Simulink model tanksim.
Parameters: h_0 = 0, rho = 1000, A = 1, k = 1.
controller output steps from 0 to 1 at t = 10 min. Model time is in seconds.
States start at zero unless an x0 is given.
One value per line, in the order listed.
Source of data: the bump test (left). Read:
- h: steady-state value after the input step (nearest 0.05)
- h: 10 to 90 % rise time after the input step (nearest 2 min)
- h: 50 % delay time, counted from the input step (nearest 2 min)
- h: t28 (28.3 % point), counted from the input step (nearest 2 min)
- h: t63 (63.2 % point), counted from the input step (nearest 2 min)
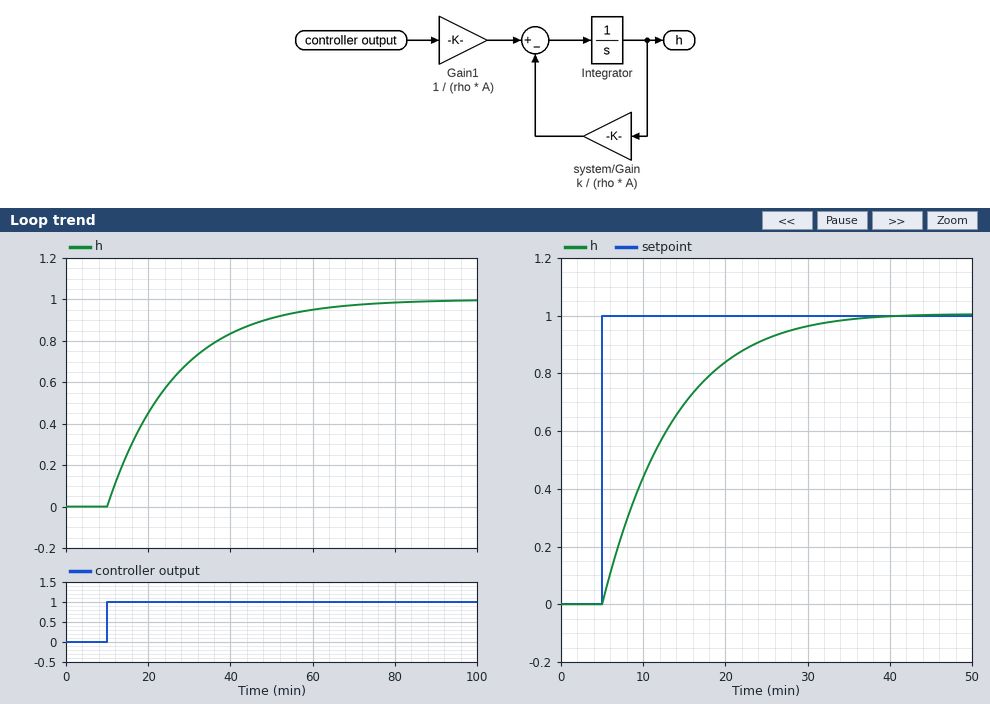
1.00
36 min
12 min
6 min
16 min
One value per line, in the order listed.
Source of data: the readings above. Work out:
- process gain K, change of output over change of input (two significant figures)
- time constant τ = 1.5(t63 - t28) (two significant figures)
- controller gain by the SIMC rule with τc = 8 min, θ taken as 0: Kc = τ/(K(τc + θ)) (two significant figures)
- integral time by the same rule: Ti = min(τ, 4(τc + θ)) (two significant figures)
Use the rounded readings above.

1.0
15 min
1.9
15 min
